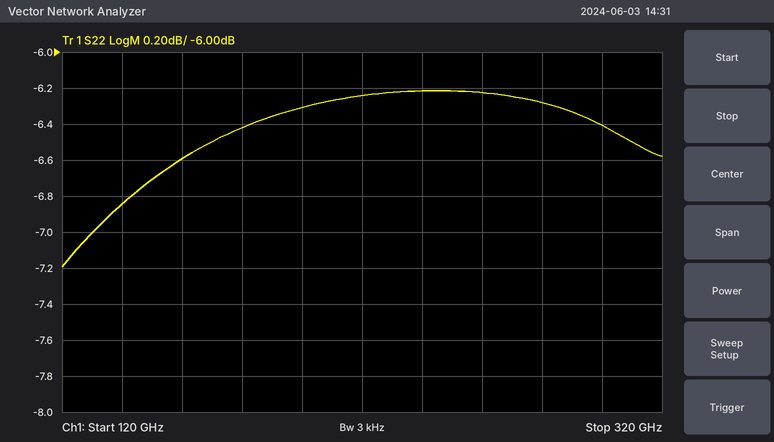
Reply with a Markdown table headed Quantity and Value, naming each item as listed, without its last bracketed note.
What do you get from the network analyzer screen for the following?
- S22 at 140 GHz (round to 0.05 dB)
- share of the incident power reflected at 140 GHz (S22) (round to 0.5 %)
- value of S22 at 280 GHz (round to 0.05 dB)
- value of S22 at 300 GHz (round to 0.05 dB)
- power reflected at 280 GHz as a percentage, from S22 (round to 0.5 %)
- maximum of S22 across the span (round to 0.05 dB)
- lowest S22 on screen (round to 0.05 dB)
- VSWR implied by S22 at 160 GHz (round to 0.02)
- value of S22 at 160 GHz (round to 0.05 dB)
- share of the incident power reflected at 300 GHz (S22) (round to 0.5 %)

| Quantity | Value |
|---|---|
| S22 at 140 GHz | -6.85 dB |
| share of the incident power reflected at 140 GHz (S22) | 20.5 % |
| value of S22 at 280 GHz | -6.30 dB |
| value of S22 at 300 GHz | -6.40 dB |
| power reflected at 280 GHz as a percentage, from S22 | 23.5 % |
| maximum of S22 across the span | -6.20 dB |
| lowest S22 on screen | -7.20 dB |
| VSWR implied by S22 at 160 GHz | 2.76 |
| value of S22 at 160 GHz | -6.60 dB |
| share of the incident power reflected at 300 GHz (S22) | 23.0 % |
